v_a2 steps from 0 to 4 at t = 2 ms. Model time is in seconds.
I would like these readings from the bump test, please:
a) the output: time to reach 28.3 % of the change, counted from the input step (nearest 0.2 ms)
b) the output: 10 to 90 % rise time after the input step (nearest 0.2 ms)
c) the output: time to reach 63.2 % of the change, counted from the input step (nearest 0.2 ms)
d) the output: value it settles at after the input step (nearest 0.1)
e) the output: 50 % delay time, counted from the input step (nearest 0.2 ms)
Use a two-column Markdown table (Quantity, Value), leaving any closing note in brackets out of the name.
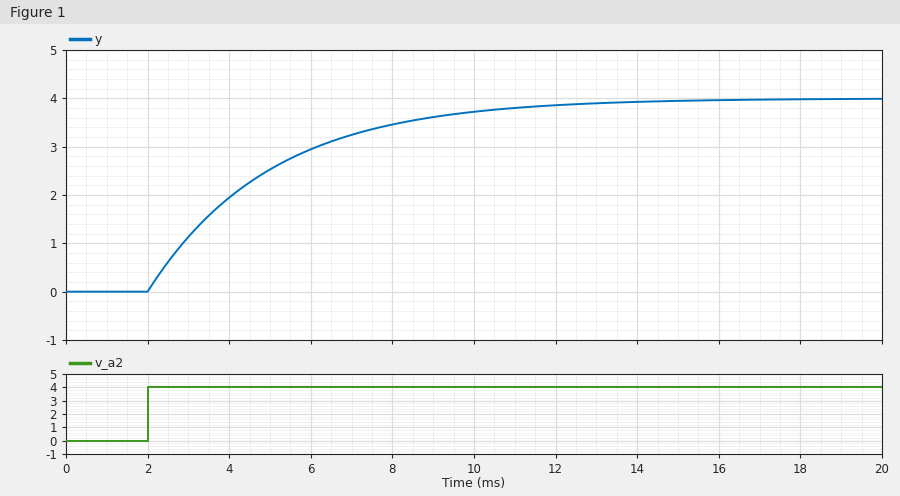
| Quantity | Value |
|---|---|
| the output: time to reach 28.3 % of the change, counted from the input step | 1.0 ms |
| the output: 10 to 90 % rise time after the input step | 6.6 ms |
| the output: time to reach 63.2 % of the change, counted from the input step | 3.0 ms |
| the output: value it settles at after the input step | 4.0 |
| the output: 50 % delay time, counted from the input step | 2.0 ms |
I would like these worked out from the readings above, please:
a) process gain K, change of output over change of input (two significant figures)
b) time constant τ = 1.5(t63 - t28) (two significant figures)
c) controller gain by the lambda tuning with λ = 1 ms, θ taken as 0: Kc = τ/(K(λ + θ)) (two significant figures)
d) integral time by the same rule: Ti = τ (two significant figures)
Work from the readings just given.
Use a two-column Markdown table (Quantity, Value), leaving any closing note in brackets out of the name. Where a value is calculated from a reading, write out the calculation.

| Quantity | Value |
|---|---|
| process gain K, change of output over change of input | (4 - 0) / 4 = 1.0 |
| time constant τ = 1.5(t63 - t28) | 1.5 × (3 - 1) = 3.0 ms |
| controller gain by the lambda tuning with λ = 1 ms, θ taken as 0: Kc = τ/(K(λ + θ)) | 3 / (1 × (1 + 0)) = 3.0 |
| integral time by the same rule: Ti = τ | 3.0 ms |
